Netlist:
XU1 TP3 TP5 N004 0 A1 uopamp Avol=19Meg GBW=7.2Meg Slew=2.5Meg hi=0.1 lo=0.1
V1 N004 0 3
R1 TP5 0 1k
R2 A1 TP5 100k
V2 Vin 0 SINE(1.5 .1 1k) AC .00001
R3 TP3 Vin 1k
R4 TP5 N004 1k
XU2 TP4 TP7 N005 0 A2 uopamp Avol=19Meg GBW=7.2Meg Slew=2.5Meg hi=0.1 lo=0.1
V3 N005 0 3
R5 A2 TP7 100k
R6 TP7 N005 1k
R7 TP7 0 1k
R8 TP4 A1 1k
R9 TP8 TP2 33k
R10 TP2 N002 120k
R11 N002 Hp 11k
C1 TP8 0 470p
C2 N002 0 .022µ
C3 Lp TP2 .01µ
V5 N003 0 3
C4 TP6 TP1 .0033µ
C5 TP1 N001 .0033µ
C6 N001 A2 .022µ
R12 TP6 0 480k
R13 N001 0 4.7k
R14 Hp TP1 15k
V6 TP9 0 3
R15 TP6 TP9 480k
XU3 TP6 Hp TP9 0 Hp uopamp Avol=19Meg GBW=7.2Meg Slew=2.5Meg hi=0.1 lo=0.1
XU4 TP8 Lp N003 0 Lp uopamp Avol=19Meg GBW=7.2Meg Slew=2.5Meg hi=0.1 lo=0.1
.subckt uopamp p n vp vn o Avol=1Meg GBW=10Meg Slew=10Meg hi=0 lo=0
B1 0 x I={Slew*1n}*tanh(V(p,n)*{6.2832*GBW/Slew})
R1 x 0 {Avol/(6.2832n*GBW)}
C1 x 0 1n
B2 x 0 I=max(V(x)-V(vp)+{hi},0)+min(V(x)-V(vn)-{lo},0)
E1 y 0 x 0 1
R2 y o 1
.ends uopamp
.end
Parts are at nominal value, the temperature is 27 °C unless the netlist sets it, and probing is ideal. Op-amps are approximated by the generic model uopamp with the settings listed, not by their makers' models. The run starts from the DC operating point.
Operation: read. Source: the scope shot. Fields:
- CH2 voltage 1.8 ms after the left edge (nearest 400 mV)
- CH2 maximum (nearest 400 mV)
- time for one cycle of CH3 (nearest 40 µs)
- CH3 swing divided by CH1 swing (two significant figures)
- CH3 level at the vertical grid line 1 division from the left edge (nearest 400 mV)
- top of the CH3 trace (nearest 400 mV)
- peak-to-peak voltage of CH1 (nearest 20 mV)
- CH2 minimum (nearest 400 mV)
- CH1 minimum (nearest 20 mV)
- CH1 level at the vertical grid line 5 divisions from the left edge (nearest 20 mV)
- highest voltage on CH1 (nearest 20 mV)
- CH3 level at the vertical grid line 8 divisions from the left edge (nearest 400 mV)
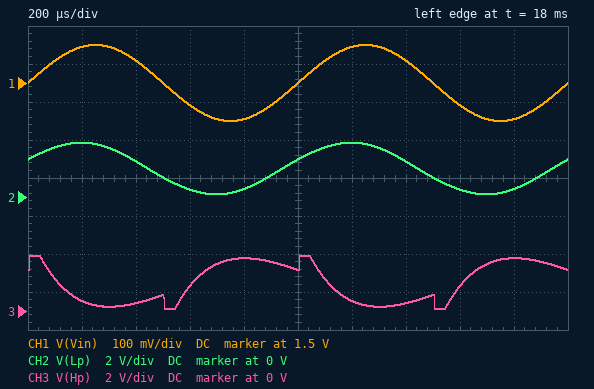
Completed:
400 mV
2.8 V
1.00 ms
14
400 mV
2.8 V
200 mV
0 V
1.40 V
1.50 V
1.60 V
1.2 V
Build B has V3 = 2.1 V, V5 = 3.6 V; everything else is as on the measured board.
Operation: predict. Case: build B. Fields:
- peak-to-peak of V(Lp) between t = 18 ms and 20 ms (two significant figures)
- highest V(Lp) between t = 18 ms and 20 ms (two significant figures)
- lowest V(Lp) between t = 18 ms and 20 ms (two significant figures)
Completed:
2.0 V
2.5 V
520 mV
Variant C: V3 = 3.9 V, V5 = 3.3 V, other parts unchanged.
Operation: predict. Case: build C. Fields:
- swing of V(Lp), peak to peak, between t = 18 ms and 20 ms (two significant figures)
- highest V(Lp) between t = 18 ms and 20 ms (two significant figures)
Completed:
2.9 V
3.0 V
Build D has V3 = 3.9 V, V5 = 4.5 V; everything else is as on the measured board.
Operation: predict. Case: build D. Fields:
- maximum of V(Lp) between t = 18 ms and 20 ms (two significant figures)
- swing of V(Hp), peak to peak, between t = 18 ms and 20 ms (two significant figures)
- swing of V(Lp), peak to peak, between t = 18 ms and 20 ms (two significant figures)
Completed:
3.0 V
2.8 V
2.9 V
